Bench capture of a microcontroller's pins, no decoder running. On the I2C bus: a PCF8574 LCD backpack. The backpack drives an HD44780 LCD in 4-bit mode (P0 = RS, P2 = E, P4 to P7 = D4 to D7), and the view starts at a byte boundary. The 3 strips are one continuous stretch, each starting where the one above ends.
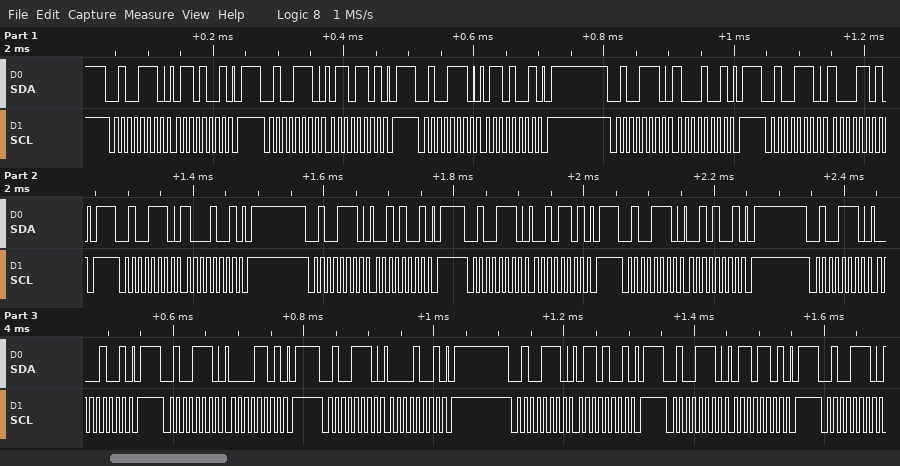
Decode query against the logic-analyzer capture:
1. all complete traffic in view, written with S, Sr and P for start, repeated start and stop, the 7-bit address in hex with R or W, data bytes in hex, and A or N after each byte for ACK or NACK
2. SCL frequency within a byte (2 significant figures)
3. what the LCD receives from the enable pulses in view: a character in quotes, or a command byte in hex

S 27W A 69 A P S 27W A 6D A P S 27W A 69 A P S 27W A 89 A P S 27W A 8D A P S 27W A 89 A P S 27W A 29 A P S 27W A 2D A P S 27W A 29 A P S 27W A 09 A P S 27W A 0D A P S 27W A 09 A P S 27W A 69 A P S 27W A 6D A P S 27W A
100 kHz
'h' ' '
